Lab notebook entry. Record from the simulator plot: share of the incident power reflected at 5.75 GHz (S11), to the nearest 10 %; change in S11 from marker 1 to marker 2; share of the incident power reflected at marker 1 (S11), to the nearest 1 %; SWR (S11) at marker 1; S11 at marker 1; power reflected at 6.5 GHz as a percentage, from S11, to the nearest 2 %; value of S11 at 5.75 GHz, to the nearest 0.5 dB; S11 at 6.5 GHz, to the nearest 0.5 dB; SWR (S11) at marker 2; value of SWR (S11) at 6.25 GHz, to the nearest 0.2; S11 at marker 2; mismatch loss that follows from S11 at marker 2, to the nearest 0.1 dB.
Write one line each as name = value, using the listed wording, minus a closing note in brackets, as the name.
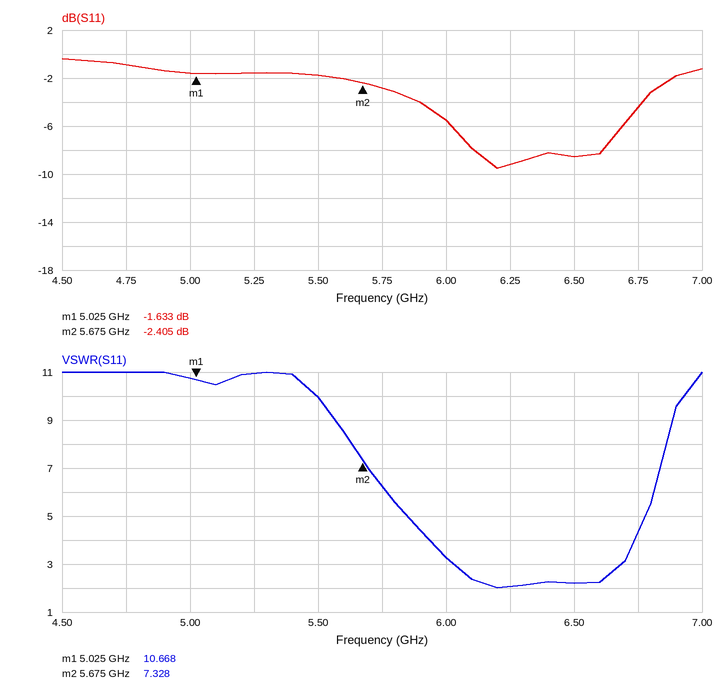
share of the incident power reflected at 5.75 GHz (S11), to the nearest 10 % = 50 %
change in S11 from marker 1 to marker 2 = -0.772 dB
share of the incident power reflected at marker 1 (S11), to the nearest 1 % = 69 %
SWR (S11) at marker 1 = 10.668
S11 at marker 1 = -1.633 dB
power reflected at 6.5 GHz as a percentage, from S11, to the nearest 2 % = 14 %
value of S11 at 5.75 GHz, to the nearest 0.5 dB = -3.0 dB
S11 at 6.5 GHz, to the nearest 0.5 dB = -8.5 dB
SWR (S11) at marker 2 = 7.328
value of SWR (S11) at 6.25 GHz, to the nearest 0.2 = 2.0
S11 at marker 2 = -2.405 dB
mismatch loss that follows from S11 at marker 2, to the nearest 0.1 dB = 3.7 dB
